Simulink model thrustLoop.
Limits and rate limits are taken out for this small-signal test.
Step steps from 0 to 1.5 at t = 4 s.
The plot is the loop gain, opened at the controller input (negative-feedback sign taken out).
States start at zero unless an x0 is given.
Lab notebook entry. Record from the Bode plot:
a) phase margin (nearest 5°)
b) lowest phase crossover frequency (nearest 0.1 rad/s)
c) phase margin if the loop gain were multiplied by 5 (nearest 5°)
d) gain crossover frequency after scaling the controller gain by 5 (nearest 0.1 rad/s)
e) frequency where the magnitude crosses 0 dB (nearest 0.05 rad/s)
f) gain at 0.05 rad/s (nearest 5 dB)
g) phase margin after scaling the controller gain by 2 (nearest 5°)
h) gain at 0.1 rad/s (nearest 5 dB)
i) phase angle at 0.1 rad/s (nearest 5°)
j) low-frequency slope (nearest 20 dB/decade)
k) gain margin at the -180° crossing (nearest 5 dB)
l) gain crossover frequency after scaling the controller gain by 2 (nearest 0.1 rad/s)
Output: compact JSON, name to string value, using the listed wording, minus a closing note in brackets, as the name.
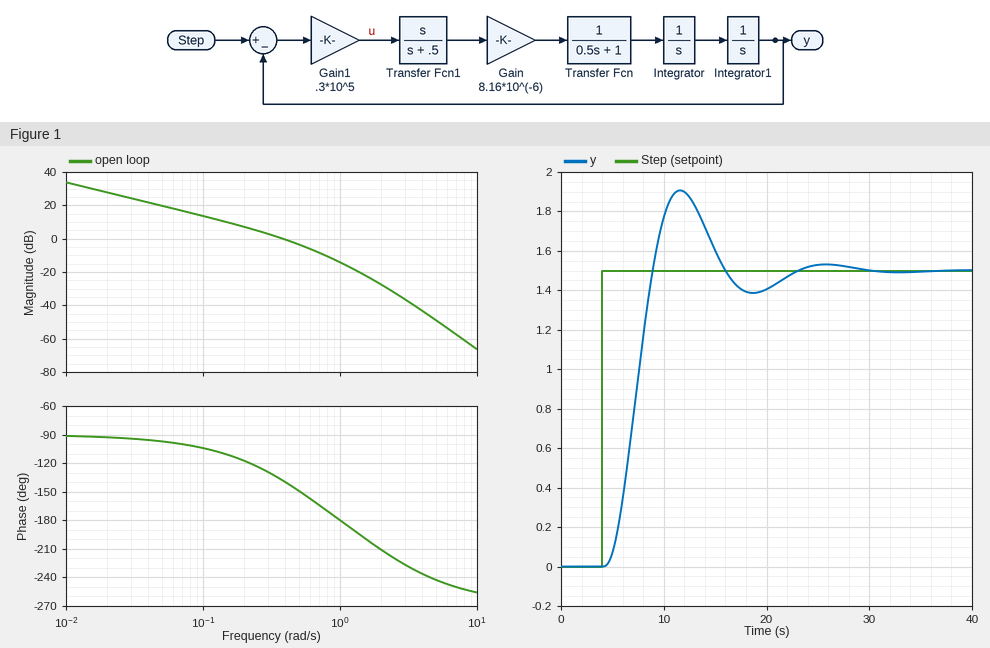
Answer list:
{"phase margin": "40°", "lowest phase crossover frequency": "1.0 rad/s", "phase margin if the loop gain were multiplied by 5": "0°", "gain crossover frequency after scaling the controller gain by 5": "1.0 rad/s", "frequency where the magnitude crosses 0 dB": "0.40 rad/s", "gain at 0.05 rad/s": "20 dB", "phase margin after scaling the controller gain by 2": "25°", "gain at 0.1 rad/s": "15 dB", "phase angle at 0.1 rad/s": "-105°", "low-frequency slope": "-20 dB/decade", "gain margin at the -180° crossing": "15 dB", "gain crossover frequency after scaling the controller gain by 2": "0.6 rad/s"}
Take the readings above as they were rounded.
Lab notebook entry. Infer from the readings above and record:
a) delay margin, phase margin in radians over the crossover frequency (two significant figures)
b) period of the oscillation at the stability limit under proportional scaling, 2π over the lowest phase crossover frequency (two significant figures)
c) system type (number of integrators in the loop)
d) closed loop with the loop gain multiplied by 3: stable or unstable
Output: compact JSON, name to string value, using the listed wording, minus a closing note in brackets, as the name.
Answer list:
{"delay margin, phase margin in radians over the crossover frequency": "1.7 s", "period of the oscillation at the stability limit under proportional scaling, 2π over the lowest phase crossover frequency": "6.3 s", "system type": "1", "closed loop with the loop gain multiplied by 3: stable or unstable": "stable"}
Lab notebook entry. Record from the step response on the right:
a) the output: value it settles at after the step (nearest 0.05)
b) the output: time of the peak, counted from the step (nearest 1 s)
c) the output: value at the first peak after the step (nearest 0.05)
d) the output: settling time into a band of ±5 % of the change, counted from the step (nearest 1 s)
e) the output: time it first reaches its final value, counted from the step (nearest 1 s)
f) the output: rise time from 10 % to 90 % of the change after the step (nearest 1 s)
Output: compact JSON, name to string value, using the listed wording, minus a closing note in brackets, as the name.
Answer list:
{"the output: value it settles at after the step": "1.50", "the output: time of the peak, counted from the step": "8 s", "the output: value at the first peak after the step": "1.90", "the output: settling time into a band of ±5 % of the change, counted from the step": "17 s", "the output: time it first reaches its final value, counted from the step": "5 s", "the output: rise time from 10 % to 90 % of the change after the step": "3 s"}
